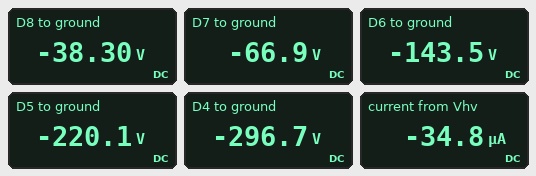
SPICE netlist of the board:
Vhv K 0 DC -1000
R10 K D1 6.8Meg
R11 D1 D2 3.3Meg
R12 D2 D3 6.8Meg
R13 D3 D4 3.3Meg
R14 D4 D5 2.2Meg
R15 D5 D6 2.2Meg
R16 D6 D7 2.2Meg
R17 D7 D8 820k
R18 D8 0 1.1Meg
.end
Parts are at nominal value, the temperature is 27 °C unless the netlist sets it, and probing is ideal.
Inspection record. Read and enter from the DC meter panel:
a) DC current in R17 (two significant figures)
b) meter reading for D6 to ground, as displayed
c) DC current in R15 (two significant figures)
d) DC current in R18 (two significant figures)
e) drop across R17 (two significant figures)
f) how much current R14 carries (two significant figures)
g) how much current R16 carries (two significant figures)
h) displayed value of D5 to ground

35 µA
-143.5 V
35 µA
35 µA
29 V
35 µA
35 µA
-220.1 V
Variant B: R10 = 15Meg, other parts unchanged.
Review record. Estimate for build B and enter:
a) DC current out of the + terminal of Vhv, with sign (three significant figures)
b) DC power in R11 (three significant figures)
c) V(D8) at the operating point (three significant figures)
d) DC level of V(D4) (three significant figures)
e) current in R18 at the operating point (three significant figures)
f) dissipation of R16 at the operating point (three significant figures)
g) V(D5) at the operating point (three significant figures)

-27.1 µA
2.42 mW
-29.8 V
-231 V
27.1 µA
1.61 mW
-171 V
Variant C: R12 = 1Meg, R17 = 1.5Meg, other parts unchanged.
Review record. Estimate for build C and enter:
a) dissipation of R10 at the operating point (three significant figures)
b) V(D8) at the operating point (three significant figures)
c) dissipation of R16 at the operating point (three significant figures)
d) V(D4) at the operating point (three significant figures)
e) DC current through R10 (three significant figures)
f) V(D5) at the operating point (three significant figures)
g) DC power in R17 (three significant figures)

12.2 mW
-46.6 V
3.95 mW
-390 V
42.4 µA
-297 V
2.69 mW
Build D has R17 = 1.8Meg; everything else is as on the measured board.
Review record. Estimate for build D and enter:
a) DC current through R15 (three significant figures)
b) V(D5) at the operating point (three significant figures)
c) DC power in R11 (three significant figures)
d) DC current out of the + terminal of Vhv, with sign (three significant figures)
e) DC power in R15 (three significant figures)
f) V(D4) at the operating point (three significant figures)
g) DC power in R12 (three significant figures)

33.7 µA
-246 V
3.74 mW
-33.7 µA
2.49 mW
-320 V
7.71 mW
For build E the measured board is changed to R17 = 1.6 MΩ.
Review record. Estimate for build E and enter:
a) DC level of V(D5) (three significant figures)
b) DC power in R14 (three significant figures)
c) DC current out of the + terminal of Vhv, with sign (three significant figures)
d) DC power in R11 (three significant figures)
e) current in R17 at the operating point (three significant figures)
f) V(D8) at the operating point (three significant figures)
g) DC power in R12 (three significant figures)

-241 V
2.53 mW
-33.9 µA
3.79 mW
33.9 µA
-37.3 V
7.81 mW
